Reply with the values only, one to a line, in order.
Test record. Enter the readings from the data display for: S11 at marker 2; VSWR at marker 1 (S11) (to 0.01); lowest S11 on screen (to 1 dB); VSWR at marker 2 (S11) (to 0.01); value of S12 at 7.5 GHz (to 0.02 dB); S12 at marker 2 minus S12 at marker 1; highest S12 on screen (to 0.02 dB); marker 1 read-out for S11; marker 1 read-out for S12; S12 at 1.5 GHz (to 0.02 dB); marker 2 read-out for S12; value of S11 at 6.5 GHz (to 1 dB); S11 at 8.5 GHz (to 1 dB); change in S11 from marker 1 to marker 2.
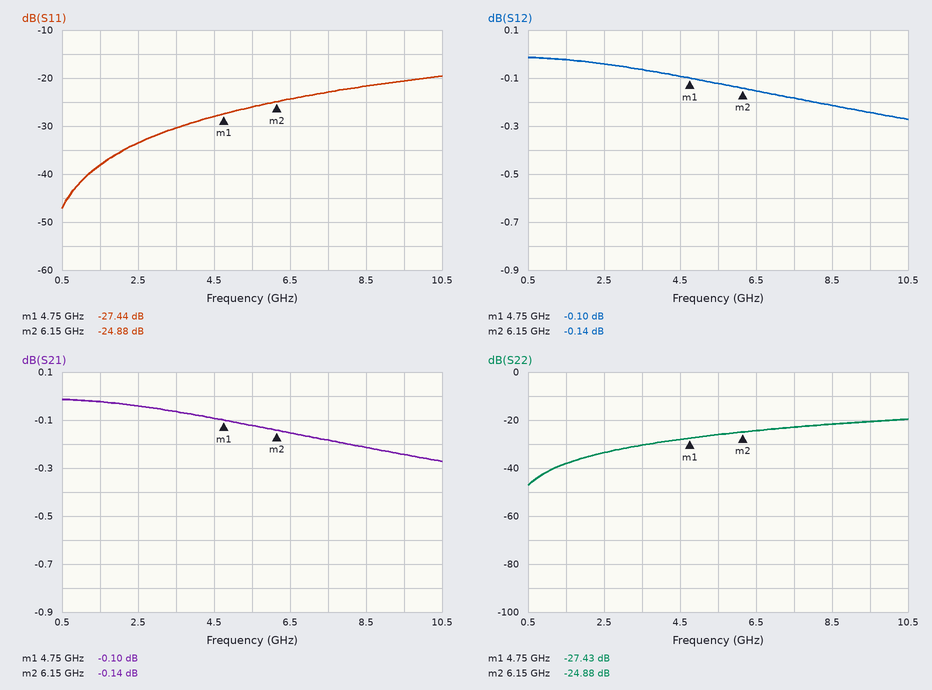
-24.88 dB
1.09
-47 dB
1.12
-0.18 dB
-0.04 dB
-0.02 dB
-27.44 dB
-0.10 dB
-0.02 dB
-0.14 dB
-24 dB
-22 dB
2.56 dB
